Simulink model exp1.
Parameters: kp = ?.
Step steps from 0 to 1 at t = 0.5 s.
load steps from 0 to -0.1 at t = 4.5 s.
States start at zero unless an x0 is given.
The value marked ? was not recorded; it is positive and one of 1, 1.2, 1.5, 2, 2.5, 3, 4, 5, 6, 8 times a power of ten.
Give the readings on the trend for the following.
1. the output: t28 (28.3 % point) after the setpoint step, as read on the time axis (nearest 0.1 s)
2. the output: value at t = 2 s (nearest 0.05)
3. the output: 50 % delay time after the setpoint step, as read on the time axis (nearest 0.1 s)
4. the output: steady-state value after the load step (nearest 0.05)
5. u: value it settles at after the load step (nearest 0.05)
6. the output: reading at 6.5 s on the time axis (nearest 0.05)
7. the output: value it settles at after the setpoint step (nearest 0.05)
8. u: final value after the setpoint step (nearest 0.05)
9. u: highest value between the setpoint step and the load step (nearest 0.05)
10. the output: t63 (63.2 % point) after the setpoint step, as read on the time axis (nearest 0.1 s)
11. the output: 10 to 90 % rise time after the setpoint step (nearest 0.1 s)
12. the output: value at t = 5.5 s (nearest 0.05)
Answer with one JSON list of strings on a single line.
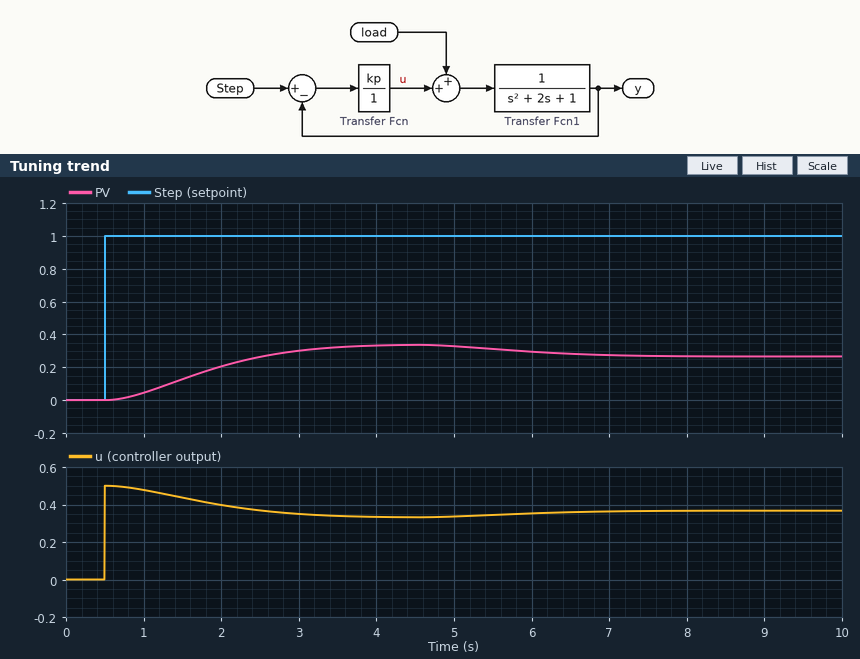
["1.3 s", "0.20", "1.7 s", "0.25", "0.35", "0.30", "0.35", "0.35", "0.50", "2.0 s", "2.1 s", "0.30"]
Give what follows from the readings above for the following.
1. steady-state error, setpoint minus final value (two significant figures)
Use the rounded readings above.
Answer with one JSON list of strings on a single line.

["0.65"]
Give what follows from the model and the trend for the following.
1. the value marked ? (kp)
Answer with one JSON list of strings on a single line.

["0.5"]
